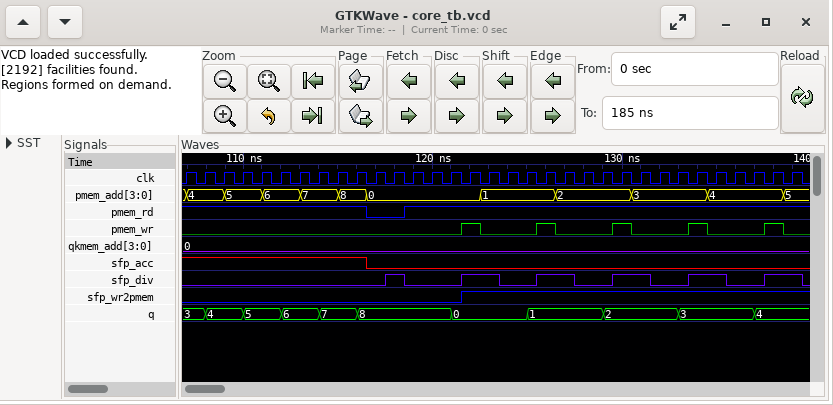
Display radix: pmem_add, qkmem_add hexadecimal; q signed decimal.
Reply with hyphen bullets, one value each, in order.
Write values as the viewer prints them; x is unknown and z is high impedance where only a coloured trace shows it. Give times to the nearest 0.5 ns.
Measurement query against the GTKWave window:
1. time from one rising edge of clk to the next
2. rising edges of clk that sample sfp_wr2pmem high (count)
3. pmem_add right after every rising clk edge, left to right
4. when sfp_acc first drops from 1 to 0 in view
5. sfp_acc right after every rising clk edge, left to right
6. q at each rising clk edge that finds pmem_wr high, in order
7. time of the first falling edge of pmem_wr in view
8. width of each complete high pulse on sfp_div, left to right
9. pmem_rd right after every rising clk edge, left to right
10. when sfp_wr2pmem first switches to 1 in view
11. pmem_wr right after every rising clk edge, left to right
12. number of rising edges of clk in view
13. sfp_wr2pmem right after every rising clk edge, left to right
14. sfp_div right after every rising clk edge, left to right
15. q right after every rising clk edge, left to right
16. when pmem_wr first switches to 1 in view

- 1 ns
- 18
- 4, 4, 5, 5, 6, 6, 7, 7, 8, 8, 0, 0, 0, 0, 0, 0, 1, 1, 1, 1, 2, 2, 2, 2, 3, 3, 3, 3, 4, 4, 4, 4, 5
- 116.5 ns
- 1 1 1 1 1 1 1 1 1 1 0 0 0 0 0 0 0 0 0 0 0 0 0 0 0 0 0 0 0 0 0 0 0
- 0, 1, 2, 3, 4
- 122.5 ns
- 1 ns, 2 ns, 2 ns, 2 ns, 2 ns, 2 ns
- 1 1 1 1 1 1 1 1 1 1 0 0 1 1 1 1 1 1 1 1 1 1 1 1 1 1 1 1 1 1 1 1 1
- 121.5 ns
- 0 0 0 0 0 0 0 0 0 0 0 0 0 0 0 1 0 0 0 1 0 0 0 1 0 0 0 1 0 0 0 1 0
- 33
- 0 0 0 0 0 0 0 0 0 0 0 0 0 0 0 1 1 1 1 1 1 1 1 1 1 1 1 1 1 1 1 1 1
- 0 0 0 0 0 0 0 0 0 0 0 1 0 0 0 1 1 0 0 1 1 0 0 1 1 0 0 1 1 0 0 1 1
- 3, 4, 4, 5, 5, 6, 6, 7, 7, 8, 8, 8, 8, 8, 0, 0, 0, 0, 1, 1, 1, 1, 2, 2, 2, 2, 3, 3, 3, 3, 4, 4, 4
- 121.5 ns
